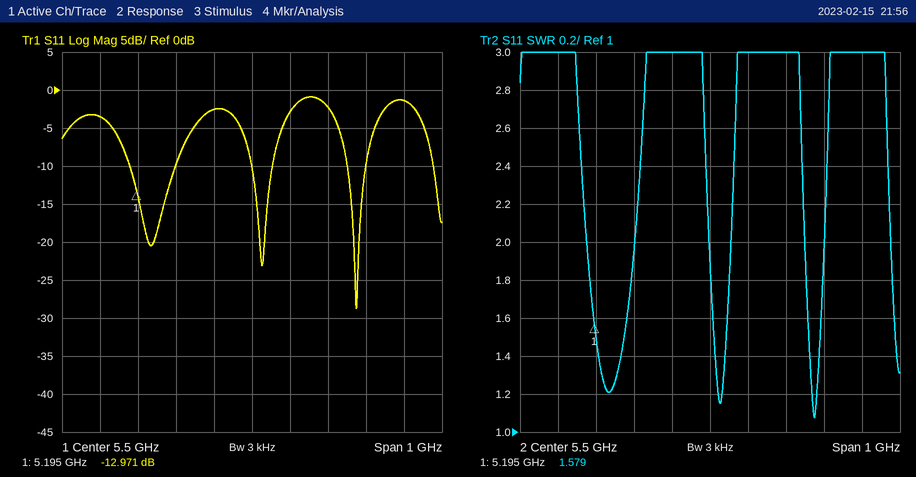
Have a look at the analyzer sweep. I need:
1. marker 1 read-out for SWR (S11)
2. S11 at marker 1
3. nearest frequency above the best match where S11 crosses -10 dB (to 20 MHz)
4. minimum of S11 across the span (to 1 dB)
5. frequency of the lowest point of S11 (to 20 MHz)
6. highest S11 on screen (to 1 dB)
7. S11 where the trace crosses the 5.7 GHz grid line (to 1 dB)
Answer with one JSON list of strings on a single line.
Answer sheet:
["1.579", "-12.971 dB", "5.80 GHz", "-29 dB", "5.78 GHz", "-1 dB", "-2 dB"]
